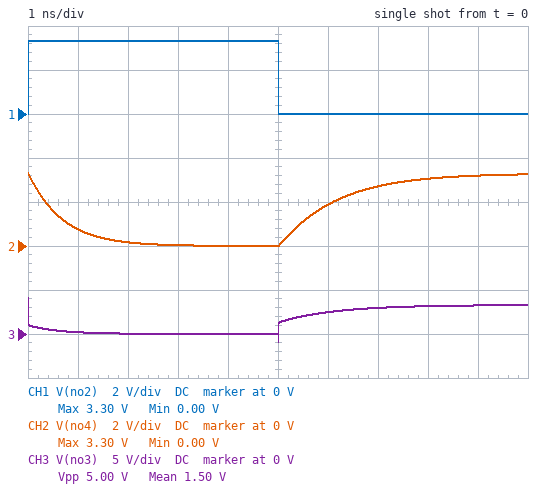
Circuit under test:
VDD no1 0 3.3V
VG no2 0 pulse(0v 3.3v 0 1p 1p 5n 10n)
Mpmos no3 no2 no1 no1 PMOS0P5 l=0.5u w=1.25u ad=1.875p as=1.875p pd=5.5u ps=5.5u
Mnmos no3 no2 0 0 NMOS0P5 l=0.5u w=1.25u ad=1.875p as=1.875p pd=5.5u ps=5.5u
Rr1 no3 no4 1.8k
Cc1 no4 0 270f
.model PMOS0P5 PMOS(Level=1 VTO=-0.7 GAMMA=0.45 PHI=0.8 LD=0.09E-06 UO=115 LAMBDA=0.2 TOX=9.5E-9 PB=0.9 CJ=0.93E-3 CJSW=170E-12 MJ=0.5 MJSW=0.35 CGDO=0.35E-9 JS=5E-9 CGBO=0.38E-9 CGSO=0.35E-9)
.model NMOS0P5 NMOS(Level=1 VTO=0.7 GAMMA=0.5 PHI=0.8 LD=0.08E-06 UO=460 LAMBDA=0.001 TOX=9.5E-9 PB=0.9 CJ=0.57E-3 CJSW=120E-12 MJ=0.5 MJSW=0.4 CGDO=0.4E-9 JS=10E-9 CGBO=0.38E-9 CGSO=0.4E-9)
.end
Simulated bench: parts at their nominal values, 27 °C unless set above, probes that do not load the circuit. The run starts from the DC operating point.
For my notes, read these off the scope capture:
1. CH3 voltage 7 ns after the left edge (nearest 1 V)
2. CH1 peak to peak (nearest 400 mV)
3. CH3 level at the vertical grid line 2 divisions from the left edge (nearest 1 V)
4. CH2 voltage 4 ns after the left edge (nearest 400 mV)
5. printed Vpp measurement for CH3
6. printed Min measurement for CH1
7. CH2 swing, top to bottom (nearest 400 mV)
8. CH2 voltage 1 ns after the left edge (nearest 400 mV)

3 V
3.2 V
0 V
0 V
5.00 V
0.00 V
3.2 V
800 mV
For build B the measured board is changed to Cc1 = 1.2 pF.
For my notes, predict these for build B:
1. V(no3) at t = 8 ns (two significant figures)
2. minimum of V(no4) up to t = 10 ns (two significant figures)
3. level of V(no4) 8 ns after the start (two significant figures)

2.4 V
620 mV
1.8 V
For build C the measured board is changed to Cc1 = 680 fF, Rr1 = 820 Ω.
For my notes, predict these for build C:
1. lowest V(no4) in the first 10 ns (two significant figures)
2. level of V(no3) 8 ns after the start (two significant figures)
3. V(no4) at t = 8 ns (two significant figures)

21 mV
2.6 V
2.4 V
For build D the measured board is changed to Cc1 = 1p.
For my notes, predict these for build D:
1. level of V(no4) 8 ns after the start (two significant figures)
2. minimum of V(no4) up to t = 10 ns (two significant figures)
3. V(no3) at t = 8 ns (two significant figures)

1.9 V
440 mV
2.5 V
